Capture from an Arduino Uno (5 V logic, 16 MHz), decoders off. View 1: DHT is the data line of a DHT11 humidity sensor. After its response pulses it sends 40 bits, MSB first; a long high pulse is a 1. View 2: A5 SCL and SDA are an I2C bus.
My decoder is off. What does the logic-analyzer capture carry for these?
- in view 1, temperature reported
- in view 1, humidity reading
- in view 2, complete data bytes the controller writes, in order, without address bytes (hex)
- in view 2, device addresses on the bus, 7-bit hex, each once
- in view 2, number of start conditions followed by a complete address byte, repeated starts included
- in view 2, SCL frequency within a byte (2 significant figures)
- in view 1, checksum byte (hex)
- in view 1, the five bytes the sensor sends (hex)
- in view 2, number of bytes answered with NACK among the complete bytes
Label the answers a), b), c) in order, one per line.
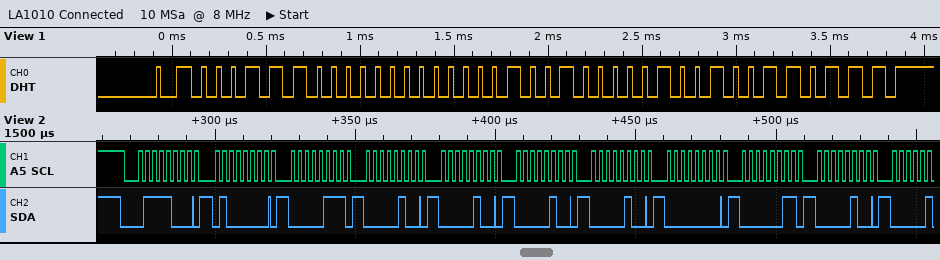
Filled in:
a) 18.9 °C
b) 28 %
c) 40 07 04 04 04 04 00 03 04
d) 0x3C
e) 1
f) 400 kHz
g) 0x37
h) 1C 00 12 09 37
i) 0
